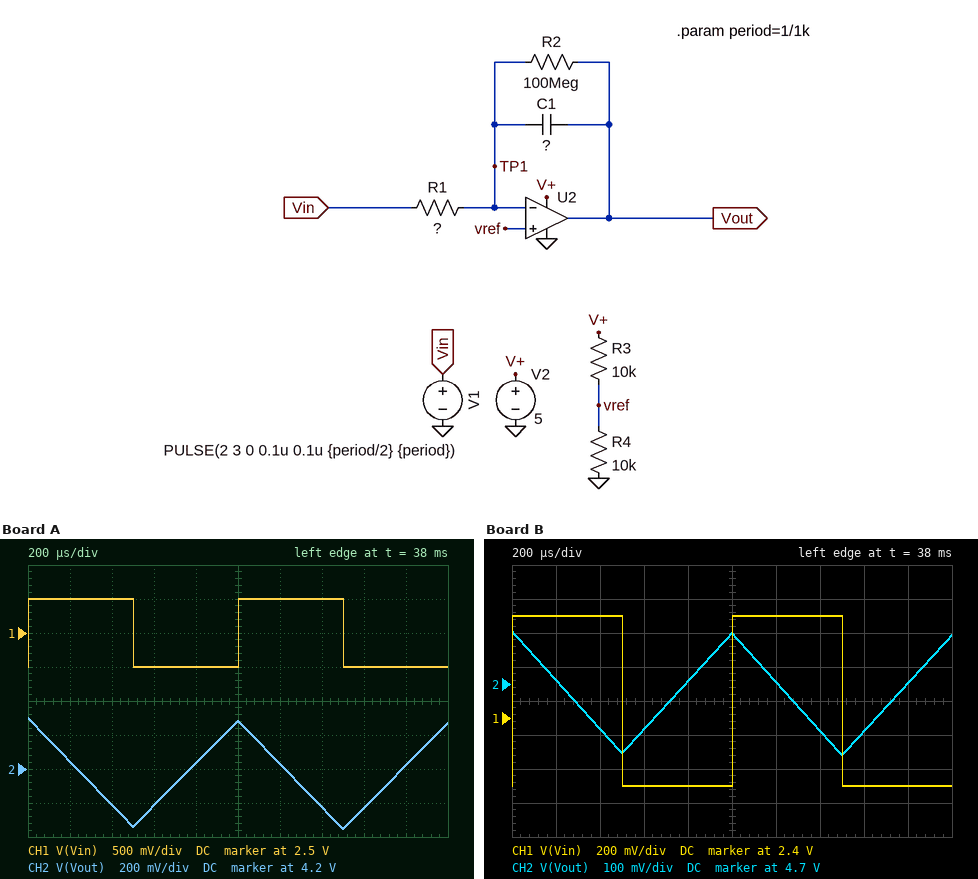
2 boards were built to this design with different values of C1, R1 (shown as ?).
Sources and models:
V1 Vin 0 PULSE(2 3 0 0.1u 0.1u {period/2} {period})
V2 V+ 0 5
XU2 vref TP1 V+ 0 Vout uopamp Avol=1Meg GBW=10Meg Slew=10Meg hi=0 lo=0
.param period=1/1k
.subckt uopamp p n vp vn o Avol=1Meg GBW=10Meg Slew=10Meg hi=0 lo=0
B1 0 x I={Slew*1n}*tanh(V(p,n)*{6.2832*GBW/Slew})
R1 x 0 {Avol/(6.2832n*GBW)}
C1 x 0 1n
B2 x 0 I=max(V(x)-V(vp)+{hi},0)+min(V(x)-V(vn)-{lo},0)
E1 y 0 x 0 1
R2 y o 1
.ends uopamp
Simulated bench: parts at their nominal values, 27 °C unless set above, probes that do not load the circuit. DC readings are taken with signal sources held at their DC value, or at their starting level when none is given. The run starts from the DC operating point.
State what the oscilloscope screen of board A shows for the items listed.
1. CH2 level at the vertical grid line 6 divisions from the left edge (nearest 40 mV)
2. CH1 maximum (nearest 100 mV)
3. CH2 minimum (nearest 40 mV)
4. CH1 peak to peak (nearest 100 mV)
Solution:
4.24 V
3.0 V
3.84 V
1.0 V
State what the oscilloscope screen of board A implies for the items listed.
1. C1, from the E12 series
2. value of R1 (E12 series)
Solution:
1.2 nF
330 kΩ
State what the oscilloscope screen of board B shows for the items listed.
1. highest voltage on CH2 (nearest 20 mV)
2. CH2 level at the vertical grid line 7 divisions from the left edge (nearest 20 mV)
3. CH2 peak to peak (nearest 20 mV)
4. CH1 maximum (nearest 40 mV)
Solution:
4.86 V
4.56 V
360 mV
3.00 V
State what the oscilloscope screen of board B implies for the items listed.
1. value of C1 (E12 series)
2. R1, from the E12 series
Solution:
3.9 nF
180 kΩ
